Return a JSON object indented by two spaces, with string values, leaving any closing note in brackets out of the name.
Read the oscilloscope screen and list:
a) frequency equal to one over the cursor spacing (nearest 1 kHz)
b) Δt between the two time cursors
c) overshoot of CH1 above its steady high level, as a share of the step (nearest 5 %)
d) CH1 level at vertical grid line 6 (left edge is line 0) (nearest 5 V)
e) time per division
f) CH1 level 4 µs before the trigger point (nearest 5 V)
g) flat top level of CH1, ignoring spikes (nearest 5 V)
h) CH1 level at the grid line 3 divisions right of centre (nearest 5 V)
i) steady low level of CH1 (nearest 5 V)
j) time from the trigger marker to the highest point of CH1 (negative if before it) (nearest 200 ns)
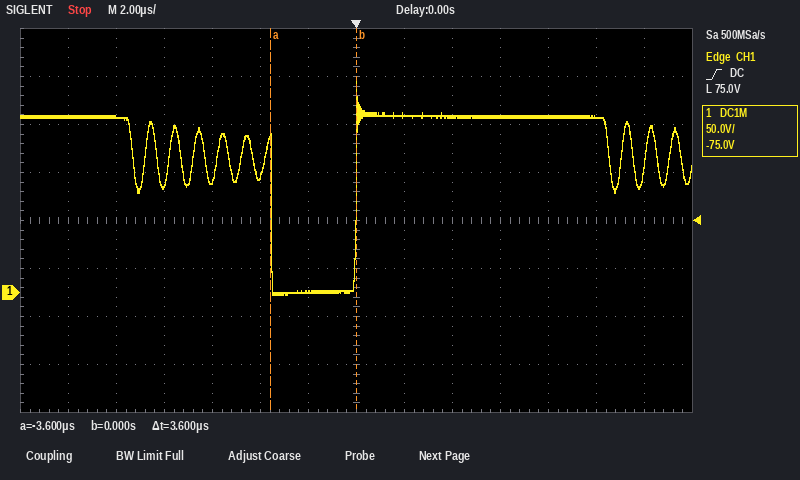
{
  "frequency equal to one over the cursor spacing": "278 kHz",
  "Δt between the two time cursors": "3.6 µs",
  "overshoot of CH1 above its steady high level, as a share of the step": "20 %",
  "CH1 level at vertical grid line 6 (left edge is line 0)": "0 V",
  "time per division": "2 µs",
  "CH1 level 4 µs before the trigger point": "120 V",
  "flat top level of CH1, ignoring spikes": "185 V",
  "CH1 level at the grid line 3 divisions right of centre": "185 V",
  "steady low level of CH1": "0 V",
  "time from the trigger marker to the highest point of CH1 (negative if before it)": "0.0 µs"
}
